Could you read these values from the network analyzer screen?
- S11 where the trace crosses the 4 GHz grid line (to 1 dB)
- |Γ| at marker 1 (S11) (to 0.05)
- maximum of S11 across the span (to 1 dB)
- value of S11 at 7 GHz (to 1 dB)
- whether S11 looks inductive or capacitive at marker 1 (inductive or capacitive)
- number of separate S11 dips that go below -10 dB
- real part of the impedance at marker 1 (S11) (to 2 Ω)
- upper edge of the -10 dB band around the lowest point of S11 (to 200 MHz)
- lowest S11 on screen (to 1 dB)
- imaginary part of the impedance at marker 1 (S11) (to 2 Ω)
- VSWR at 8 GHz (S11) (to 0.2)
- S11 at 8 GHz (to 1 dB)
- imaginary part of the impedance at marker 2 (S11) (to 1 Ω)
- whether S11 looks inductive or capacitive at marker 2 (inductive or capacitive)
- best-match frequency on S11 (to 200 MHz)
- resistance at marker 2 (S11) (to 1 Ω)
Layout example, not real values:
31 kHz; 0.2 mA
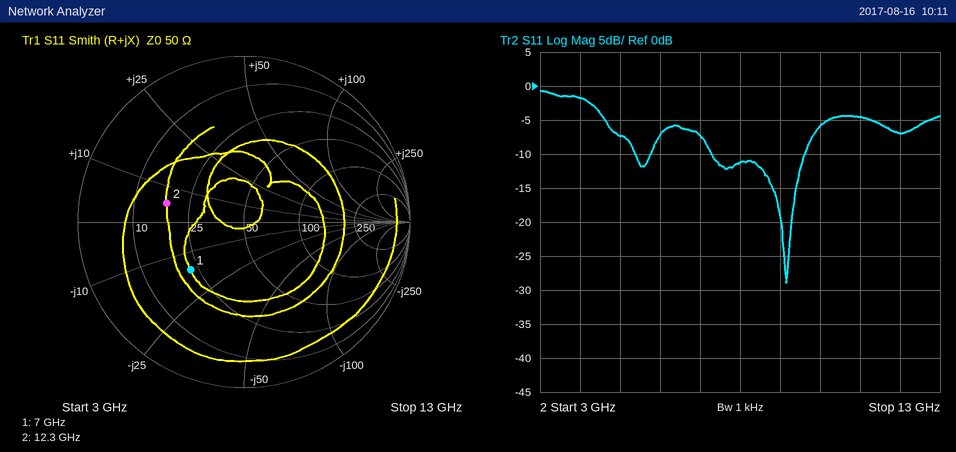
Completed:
-2 dB; 0.45; -1 dB; -7 dB; capacitive; 2; 22 Ω; 9.6 GHz; -29 dB; -16 Ω; 1.8; -11 dB; +5 Ω; inductive; 9.2 GHz; 18 Ω
